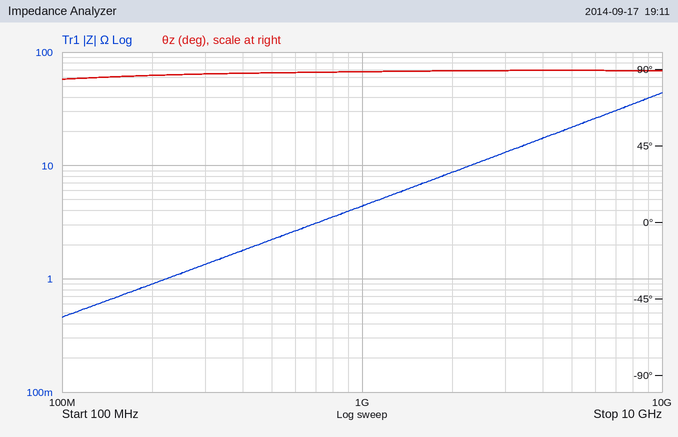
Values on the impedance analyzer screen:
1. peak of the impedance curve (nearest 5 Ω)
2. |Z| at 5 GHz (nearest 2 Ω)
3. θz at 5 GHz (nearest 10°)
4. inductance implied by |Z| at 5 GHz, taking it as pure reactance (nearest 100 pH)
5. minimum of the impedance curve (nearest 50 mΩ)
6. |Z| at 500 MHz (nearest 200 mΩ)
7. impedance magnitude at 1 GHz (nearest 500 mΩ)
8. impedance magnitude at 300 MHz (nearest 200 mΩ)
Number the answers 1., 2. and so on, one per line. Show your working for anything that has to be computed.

1. 45 Ω
2. 22 Ω
3. 90°
4. L = 22 Ω/(2π × 5 GHz) ≈ 700 pH
5. 450 mΩ
6. 2.2 Ω
7. 4.5 Ω
8. 1.4 Ω
